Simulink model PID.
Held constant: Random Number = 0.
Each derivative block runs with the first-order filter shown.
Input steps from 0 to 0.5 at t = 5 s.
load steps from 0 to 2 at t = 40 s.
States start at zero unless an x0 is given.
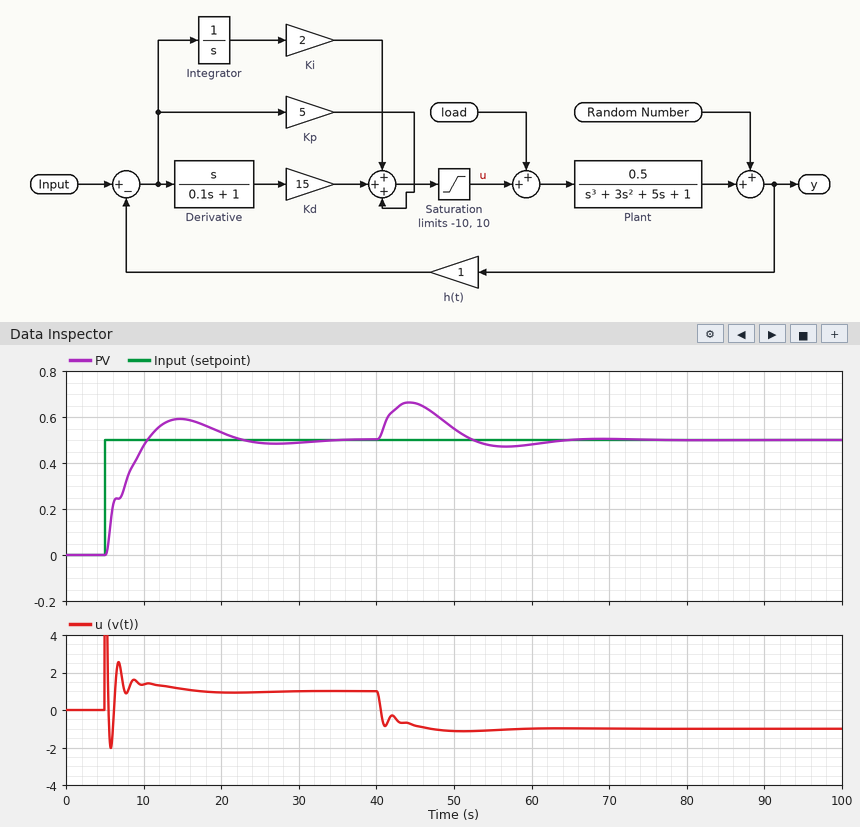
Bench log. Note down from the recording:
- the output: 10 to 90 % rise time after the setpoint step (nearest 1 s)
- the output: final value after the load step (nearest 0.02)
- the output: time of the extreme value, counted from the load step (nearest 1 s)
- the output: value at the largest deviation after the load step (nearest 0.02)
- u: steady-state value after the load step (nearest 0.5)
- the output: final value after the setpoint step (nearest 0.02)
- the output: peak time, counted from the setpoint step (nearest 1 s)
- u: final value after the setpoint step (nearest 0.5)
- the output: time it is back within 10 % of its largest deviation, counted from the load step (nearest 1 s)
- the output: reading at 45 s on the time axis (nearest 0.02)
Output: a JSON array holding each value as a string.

["4 s", "0.50", "4 s", "0.66", "-1.0", "0.50", "10 s", "1.0", "21 s", "0.66"]
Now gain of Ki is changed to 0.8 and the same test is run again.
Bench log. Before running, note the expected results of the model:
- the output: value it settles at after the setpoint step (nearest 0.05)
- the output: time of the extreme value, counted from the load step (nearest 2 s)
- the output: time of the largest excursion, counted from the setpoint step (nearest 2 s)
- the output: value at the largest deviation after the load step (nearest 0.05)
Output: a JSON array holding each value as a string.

["0.50", "6 s", "16 s", "0.70"]
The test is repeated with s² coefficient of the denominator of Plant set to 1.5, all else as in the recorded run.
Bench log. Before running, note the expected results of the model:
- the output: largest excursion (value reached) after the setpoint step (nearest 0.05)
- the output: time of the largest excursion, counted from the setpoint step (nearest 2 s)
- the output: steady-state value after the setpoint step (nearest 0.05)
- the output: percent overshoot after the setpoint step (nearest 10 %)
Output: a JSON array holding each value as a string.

["0.60", "8 s", "0.50", "20 %"]
